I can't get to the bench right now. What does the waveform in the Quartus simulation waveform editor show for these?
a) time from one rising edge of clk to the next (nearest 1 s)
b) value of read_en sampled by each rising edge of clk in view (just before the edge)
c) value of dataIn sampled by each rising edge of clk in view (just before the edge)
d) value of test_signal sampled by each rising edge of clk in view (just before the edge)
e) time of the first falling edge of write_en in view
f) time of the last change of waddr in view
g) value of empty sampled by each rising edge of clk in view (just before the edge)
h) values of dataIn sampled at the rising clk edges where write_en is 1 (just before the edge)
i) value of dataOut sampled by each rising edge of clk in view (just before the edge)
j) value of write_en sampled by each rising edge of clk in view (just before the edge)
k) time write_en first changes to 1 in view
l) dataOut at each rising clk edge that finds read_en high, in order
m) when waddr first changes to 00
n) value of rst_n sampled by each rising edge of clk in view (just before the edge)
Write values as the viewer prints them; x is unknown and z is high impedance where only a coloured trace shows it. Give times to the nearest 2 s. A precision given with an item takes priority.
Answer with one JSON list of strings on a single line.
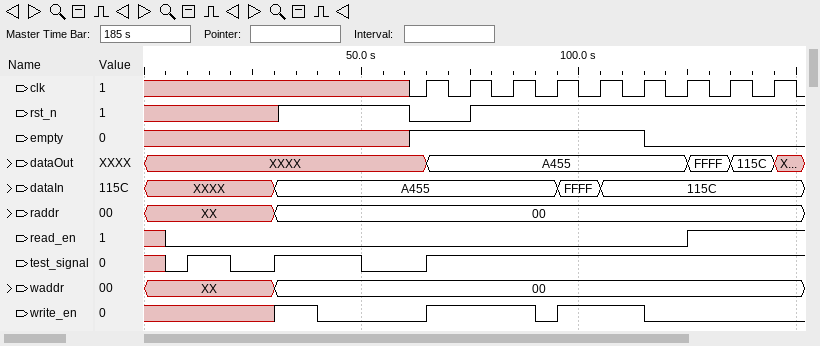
["10 s", "0 0 0 0 0 0 0 1 1", "A455, A455, A455, A455, FFFF, 115C, 115C, 115C, 115C", "0 1 1 1 1 1 1 1 1", "40 s", "30 s", "1 1 1 1 1 1 0 0 0", "A455, A455, FFFF, 115C", "XXXX, A455, A455, A455, A455, A455, A455, FFFF, 115C", "0 1 1 0 1 1 0 0 0", "30 s", "FFFF, 115C", "30 s", "0 0 1 1 1 1 1 1 1"]
